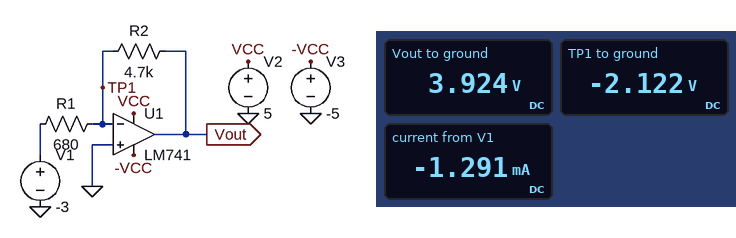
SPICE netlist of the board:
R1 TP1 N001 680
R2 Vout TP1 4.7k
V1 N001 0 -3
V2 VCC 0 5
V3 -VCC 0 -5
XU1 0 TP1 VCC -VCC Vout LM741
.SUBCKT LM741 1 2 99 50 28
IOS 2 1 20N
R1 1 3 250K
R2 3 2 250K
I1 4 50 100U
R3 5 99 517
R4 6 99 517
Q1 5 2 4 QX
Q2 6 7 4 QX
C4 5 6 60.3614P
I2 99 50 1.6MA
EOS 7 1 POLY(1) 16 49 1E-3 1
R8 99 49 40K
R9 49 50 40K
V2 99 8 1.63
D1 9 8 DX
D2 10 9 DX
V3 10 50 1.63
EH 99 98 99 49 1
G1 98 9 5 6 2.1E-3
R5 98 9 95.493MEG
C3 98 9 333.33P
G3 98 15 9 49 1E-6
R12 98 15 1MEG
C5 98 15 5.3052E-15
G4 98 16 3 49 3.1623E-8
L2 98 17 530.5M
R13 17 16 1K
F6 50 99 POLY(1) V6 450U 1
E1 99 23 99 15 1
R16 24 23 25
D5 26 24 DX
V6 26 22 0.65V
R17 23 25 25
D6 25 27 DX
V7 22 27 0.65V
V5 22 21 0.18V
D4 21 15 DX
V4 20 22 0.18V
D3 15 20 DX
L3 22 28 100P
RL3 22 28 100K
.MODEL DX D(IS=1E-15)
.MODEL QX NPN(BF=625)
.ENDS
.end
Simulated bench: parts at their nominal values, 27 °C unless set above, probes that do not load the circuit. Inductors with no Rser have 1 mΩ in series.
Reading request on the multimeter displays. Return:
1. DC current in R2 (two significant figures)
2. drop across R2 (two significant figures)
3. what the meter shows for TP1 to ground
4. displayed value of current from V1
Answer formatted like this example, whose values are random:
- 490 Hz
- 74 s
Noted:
- 1.3 mA
- 6.0 V
- -2.122 V
- -1.291 mA
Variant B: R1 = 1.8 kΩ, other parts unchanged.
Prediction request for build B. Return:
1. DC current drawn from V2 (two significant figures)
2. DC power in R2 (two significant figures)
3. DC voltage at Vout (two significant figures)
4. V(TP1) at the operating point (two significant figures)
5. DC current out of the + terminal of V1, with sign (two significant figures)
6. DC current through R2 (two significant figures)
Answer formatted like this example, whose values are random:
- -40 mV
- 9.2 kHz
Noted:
- 2.4 mA
- 5.3 mW
- 3.9 V
- -1.1 V
- -1.1 mA
- 1.1 mA
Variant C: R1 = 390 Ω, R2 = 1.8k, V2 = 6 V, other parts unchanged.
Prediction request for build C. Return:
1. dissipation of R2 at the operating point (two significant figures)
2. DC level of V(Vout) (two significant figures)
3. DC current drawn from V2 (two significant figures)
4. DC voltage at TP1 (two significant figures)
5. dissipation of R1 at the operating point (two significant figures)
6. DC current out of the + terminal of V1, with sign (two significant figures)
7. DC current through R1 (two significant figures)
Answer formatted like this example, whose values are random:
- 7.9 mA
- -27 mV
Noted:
- 23 mW
- 4.8 V
- 5.0 mA
- -1.6 V
- 5.0 mW
- -3.6 mA
- 3.6 mA
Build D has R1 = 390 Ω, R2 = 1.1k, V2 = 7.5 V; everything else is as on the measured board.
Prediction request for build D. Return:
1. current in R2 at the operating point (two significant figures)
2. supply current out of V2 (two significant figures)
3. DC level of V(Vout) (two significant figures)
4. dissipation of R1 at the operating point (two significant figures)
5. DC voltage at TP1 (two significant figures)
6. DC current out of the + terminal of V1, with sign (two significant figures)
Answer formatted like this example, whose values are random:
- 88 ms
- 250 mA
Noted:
- 6.2 mA
- 7.6 mA
- 6.3 V
- 15 mW
- -580 mV
- -6.2 mA
